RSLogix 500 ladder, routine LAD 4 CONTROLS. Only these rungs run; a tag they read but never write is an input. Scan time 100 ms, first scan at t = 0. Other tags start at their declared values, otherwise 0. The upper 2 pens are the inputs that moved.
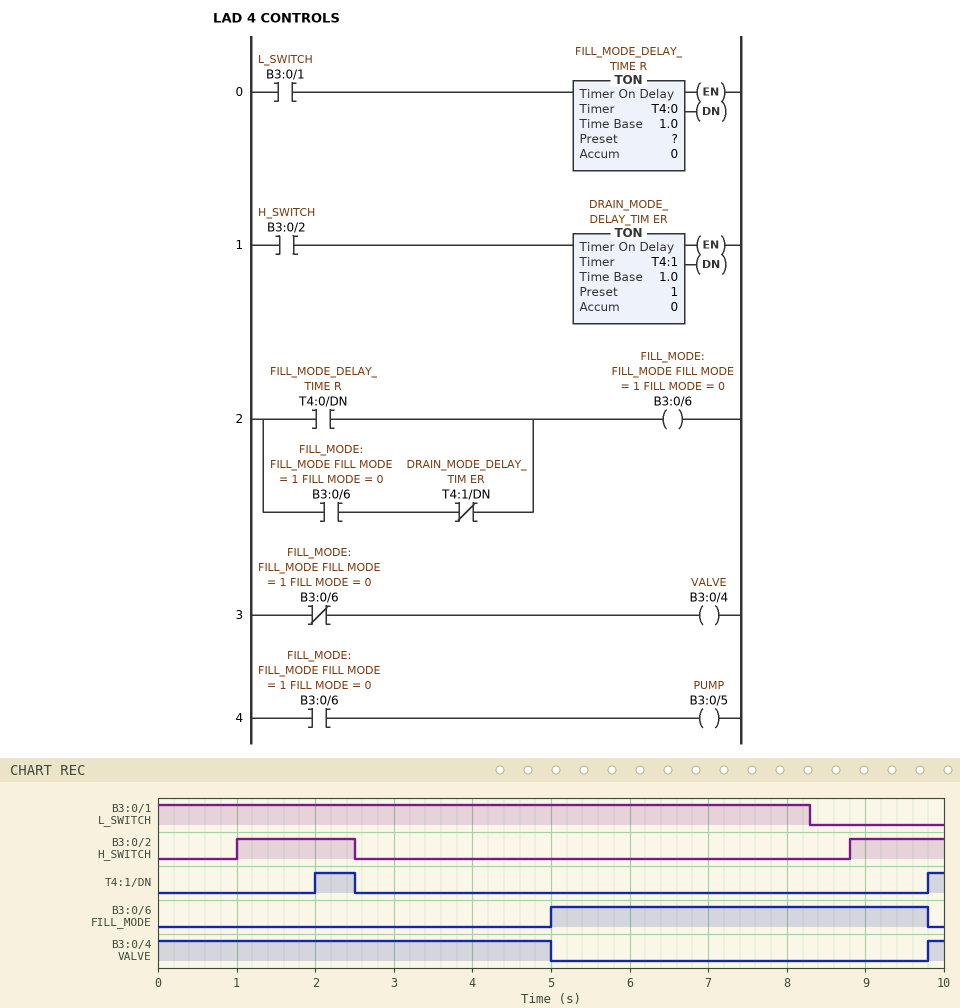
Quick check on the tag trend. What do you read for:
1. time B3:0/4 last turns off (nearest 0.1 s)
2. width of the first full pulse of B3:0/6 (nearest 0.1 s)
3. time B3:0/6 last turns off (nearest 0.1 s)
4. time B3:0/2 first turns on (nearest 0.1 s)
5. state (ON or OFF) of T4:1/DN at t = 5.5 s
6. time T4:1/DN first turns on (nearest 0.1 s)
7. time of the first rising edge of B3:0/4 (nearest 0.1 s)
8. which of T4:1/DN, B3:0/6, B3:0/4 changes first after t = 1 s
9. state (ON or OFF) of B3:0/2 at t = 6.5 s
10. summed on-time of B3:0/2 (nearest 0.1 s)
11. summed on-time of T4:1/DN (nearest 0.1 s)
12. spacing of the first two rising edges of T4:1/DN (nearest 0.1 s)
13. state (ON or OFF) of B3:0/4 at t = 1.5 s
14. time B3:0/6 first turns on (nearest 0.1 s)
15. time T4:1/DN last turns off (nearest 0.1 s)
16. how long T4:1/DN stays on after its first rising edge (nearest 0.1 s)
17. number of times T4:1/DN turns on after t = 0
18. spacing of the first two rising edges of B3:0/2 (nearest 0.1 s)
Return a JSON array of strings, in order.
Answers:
["5.0 s", "4.8 s", "9.8 s", "1.0 s", "OFF", "2.0 s", "9.8 s", "T4:1/DN", "OFF", "2.7 s", "0.7 s", "7.8 s", "ON", "5.0 s", "2.5 s", "0.5 s", "2", "7.8 s"]
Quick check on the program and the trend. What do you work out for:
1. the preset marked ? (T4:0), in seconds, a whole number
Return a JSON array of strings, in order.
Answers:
["5 s"]
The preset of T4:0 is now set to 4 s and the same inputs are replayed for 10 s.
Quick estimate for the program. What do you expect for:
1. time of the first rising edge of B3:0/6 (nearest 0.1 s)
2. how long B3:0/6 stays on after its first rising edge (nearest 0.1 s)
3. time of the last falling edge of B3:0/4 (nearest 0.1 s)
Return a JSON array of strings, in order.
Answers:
["4.0 s", "5.8 s", "4.0 s"]
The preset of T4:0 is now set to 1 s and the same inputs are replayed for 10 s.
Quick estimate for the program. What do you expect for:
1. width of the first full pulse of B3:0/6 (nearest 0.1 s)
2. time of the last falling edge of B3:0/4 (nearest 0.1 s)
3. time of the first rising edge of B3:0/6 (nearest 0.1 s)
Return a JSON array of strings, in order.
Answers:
["8.8 s", "1.0 s", "1.0 s"]
